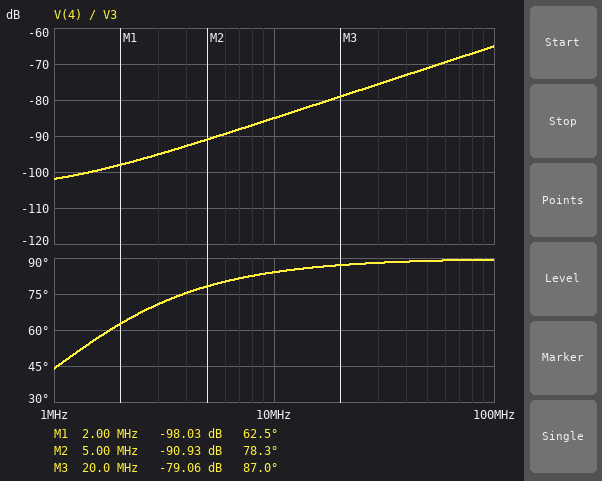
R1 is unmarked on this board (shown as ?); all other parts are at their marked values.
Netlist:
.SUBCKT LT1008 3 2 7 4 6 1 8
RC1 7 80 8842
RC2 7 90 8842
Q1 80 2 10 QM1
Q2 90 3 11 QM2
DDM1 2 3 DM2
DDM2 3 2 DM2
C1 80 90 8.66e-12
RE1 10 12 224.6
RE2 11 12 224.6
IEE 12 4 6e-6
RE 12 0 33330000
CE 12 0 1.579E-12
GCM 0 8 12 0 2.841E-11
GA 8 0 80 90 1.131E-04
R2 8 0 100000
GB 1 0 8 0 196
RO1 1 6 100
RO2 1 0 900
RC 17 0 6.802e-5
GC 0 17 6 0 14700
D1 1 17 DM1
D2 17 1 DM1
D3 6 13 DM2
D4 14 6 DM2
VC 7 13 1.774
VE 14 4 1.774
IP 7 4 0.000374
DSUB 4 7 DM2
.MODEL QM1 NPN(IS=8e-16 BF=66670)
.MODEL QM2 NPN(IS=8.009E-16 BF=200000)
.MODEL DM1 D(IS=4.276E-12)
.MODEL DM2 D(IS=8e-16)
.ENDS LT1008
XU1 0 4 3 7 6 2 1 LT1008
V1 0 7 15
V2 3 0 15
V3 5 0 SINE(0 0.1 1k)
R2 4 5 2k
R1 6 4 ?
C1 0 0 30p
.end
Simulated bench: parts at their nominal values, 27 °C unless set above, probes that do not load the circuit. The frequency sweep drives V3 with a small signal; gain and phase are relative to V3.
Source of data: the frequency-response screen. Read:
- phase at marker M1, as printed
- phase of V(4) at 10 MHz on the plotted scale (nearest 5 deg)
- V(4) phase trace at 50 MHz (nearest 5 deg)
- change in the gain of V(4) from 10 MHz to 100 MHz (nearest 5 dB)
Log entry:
62.5 deg
85 deg
90 deg
20 dB
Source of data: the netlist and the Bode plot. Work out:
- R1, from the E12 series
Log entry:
22 kΩ
